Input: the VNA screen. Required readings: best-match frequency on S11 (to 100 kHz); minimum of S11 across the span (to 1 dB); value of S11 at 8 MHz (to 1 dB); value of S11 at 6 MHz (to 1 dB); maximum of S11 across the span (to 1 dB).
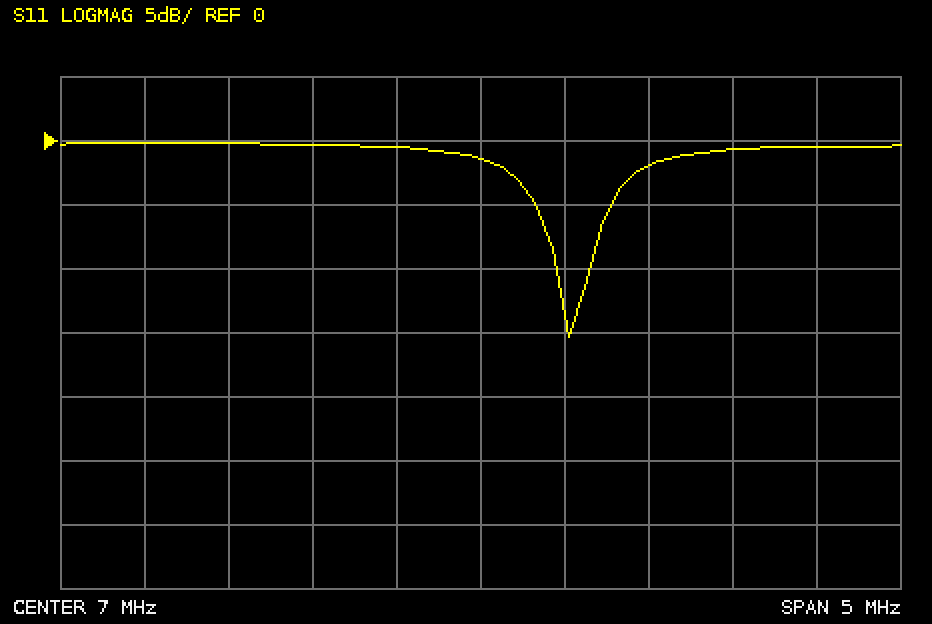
7.5 MHz
-15 dB
-2 dB
0 dB
0 dB
